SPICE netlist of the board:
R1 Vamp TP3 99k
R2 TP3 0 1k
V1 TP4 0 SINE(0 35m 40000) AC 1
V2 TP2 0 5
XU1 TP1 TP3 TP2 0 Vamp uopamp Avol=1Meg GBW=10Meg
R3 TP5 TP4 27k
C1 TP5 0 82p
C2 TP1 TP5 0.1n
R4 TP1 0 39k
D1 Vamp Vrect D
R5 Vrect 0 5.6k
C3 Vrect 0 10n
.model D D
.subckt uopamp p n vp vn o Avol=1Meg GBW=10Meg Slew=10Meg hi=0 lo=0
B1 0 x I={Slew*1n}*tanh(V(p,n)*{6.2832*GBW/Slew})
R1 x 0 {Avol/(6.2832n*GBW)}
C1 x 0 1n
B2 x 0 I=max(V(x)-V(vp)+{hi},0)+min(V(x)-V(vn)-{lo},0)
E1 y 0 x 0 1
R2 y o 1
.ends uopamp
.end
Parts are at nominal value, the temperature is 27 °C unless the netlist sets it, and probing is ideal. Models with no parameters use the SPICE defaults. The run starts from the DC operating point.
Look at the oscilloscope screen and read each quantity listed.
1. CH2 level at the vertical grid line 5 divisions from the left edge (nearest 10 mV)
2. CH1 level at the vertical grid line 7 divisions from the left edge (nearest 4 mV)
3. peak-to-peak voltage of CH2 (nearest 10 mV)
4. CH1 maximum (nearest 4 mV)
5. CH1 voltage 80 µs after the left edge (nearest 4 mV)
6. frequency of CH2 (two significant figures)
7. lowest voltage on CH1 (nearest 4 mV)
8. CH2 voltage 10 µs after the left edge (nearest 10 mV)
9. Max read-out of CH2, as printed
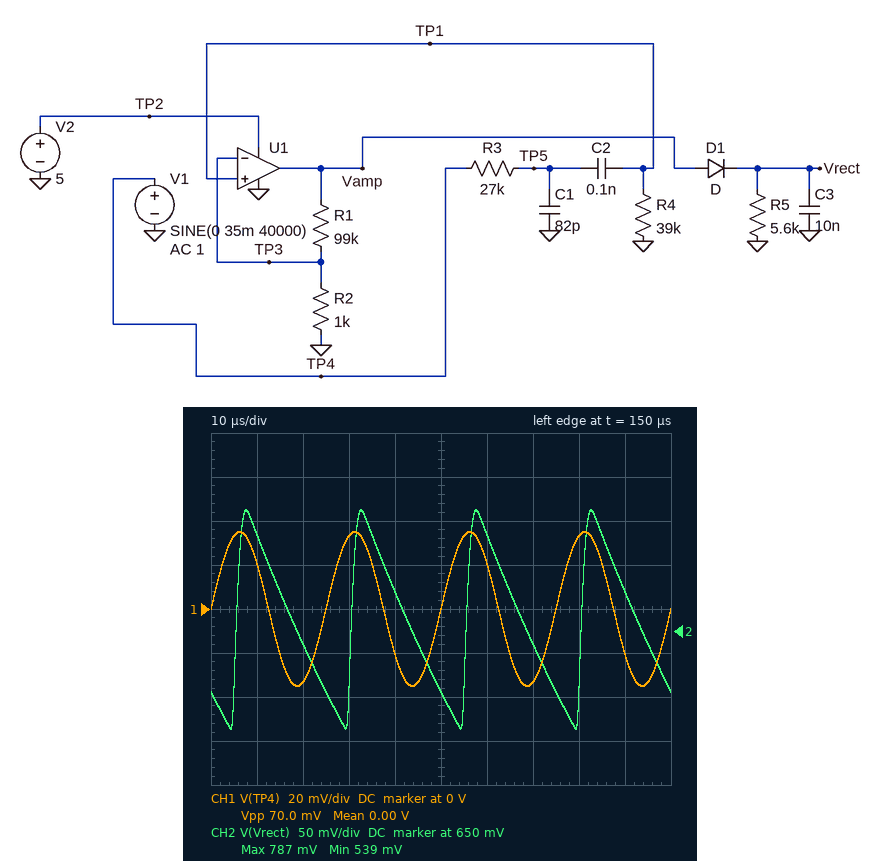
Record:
580 mV
-32 mV
250 mV
36 mV
32 mV
40 kHz
-36 mV
760 mV
787 mV
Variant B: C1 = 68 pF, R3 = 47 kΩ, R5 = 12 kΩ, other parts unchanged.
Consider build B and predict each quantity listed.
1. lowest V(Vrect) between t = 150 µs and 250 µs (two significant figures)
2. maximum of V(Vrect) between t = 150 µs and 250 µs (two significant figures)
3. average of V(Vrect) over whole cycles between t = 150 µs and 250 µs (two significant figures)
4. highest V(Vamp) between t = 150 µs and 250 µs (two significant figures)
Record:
390 mV
460 mV
420 mV
1.1 V
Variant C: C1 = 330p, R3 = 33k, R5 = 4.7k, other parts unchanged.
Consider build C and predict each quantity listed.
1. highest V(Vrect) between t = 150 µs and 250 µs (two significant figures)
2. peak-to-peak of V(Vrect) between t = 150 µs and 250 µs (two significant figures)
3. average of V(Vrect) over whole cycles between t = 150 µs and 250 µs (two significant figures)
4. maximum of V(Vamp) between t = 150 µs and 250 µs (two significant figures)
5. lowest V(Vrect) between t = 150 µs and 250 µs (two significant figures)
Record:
65 mV
23 mV
53 mV
660 mV
42 mV
